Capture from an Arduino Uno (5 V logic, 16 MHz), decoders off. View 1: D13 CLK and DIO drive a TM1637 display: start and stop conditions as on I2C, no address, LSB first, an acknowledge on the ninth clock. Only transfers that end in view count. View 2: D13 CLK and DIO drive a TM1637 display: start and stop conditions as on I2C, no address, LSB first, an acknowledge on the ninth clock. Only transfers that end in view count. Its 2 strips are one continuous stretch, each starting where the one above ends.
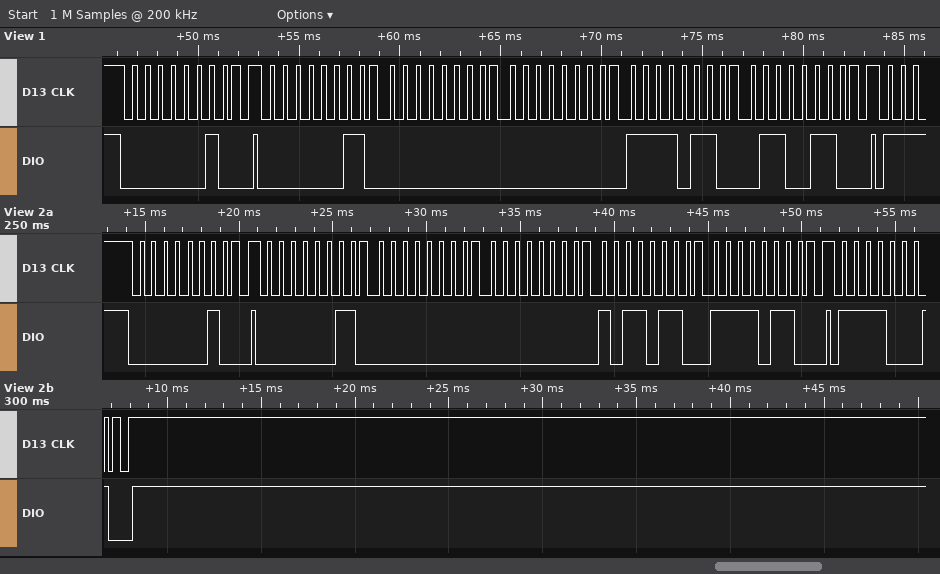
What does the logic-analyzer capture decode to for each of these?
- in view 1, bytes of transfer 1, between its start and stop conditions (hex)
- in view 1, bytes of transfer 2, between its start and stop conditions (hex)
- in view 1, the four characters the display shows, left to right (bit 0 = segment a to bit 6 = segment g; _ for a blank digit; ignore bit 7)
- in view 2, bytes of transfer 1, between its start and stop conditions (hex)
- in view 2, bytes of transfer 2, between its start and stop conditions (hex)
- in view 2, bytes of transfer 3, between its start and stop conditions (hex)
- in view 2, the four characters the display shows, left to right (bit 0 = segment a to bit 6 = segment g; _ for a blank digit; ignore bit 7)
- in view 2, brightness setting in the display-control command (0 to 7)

40
C0 00 00 6F 66
__94
40
C0 00 00 6D 6F
8F
__59
7
